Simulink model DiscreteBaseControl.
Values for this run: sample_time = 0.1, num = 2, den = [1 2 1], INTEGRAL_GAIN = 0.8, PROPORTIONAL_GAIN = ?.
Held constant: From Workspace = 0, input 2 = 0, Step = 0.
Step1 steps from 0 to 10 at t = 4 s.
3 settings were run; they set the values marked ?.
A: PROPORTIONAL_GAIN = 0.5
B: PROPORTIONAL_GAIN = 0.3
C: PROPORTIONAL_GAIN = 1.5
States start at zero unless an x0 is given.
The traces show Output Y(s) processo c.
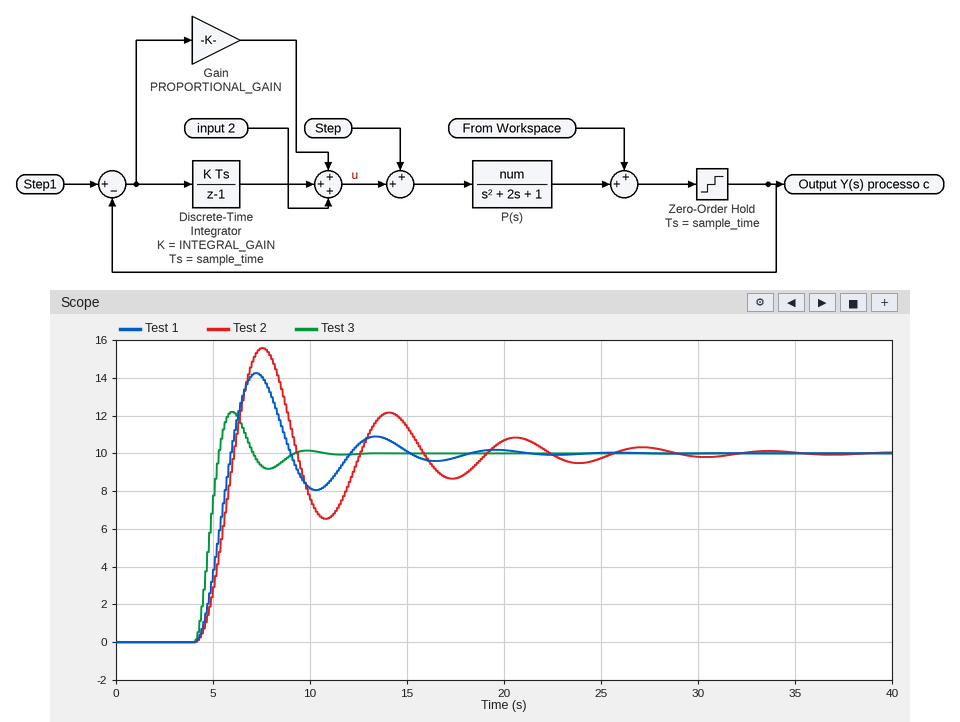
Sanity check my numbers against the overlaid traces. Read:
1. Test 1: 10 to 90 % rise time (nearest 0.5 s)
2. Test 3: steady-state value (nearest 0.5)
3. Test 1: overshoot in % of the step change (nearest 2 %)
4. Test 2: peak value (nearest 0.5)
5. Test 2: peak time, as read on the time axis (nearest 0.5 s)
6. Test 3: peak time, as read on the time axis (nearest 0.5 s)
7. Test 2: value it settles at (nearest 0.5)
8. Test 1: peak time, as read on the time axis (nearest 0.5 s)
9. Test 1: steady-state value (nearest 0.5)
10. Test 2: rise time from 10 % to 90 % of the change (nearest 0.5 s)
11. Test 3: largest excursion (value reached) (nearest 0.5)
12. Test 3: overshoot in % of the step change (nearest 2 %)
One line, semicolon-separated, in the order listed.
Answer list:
1.5 s; 10.0; 42 %; 15.5; 7.5 s; 6.0 s; 10.0; 7.0 s; 10.0; 1.5 s; 12.0; 22 %
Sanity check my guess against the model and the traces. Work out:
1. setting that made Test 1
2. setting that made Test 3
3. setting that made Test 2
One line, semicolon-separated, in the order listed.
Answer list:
A; C; B
